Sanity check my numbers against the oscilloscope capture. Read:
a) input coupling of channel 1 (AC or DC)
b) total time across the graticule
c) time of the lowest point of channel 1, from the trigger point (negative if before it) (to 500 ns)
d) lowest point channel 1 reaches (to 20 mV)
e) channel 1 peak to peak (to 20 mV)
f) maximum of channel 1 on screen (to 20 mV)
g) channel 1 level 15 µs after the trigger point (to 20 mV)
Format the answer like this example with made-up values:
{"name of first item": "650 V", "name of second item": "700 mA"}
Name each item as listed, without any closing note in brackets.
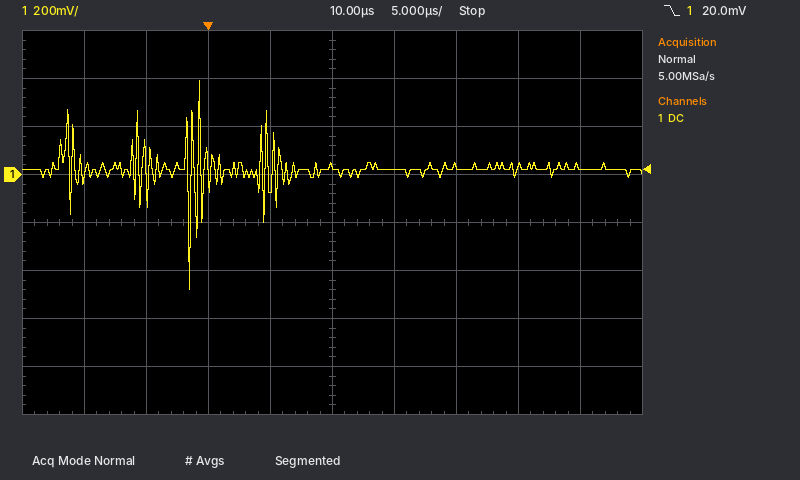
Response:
{"input coupling of channel 1": "DC", "total time across the graticule": "50 µs", "time of the lowest point of channel 1, from the trigger point (negative if before it)": "-1.5 µs", "lowest point channel 1 reaches": "-480 mV", "channel 1 peak to peak": "880 mV", "maximum of channel 1 on screen": "400 mV", "channel 1 level 15 µs after the trigger point": "20 mV"}
